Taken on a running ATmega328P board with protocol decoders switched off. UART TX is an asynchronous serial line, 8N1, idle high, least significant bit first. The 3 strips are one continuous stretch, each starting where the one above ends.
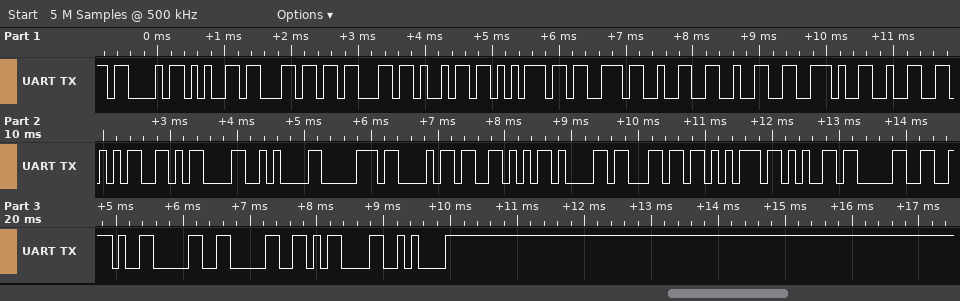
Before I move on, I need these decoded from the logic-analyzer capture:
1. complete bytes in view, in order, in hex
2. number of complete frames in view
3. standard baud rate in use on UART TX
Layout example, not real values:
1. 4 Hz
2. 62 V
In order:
1. 0x43 0x65 0x6C 0x63 0x69 0x75 0x73 0x32 0x32 0x2E 0x32 0x35 0x0D 0x0A 0x70 0x68 0x56 0x61 0x6C 0x75 0x65 0x30 0x2E 0x30 0x30 0x0D 0x0A
2. 27
3. 9600 baud
